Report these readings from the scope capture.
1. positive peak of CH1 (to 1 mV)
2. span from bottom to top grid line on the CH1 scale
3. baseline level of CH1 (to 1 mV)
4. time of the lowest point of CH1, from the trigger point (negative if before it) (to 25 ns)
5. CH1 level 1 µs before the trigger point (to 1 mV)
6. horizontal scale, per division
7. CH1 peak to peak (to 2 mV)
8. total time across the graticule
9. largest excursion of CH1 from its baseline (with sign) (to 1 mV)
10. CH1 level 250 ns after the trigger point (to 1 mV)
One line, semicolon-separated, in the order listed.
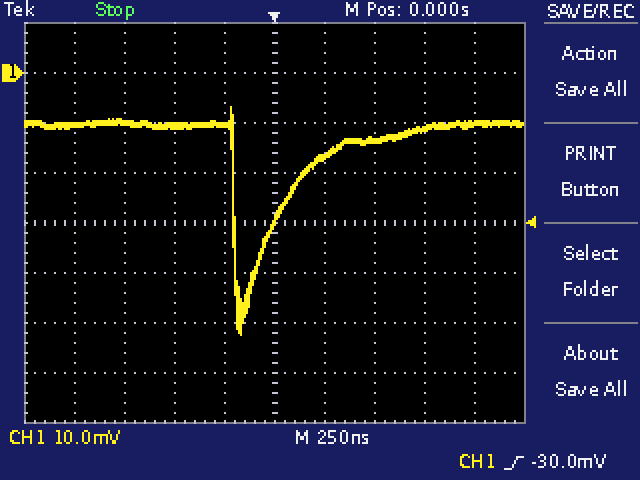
-7 mV; 80 mV; -10 mV; -175 ns; -10 mV; 250 ns; 46 mV; 2.5 µs; -42 mV; -17 mV
